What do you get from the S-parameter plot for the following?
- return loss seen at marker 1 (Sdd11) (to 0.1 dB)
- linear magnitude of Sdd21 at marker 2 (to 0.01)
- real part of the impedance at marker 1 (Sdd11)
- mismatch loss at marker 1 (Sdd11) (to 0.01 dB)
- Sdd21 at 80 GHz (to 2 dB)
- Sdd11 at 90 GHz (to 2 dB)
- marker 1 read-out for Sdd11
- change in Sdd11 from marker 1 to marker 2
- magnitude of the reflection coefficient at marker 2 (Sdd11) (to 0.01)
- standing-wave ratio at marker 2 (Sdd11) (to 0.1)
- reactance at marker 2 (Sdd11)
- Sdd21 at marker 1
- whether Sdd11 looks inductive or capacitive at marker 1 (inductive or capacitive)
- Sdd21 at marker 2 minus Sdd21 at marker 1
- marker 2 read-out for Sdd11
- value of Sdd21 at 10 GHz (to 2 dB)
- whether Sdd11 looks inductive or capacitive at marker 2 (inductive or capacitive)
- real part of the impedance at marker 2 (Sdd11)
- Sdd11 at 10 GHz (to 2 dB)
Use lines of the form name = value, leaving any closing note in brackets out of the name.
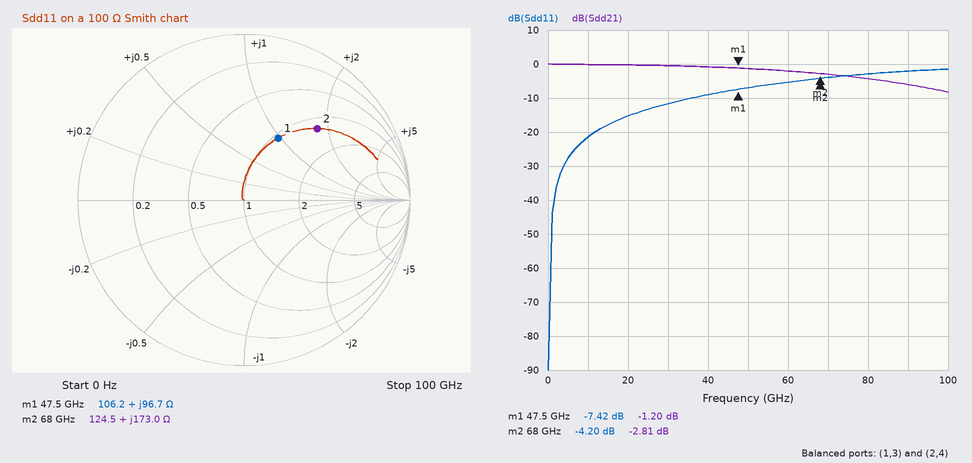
return loss seen at marker 1 (Sdd11) = 7.4 dB
linear magnitude of Sdd21 at marker 2 = 0.72
real part of the impedance at marker 1 = 106.2 Ω
mismatch loss at marker 1 (Sdd11) = 0.87 dB
Sdd21 at 80 GHz = -4 dB
Sdd11 at 90 GHz = -2 dB
marker 1 read-out for Sdd11 = -7.42 dB
change in Sdd11 from marker 1 to marker 2 = 3.22 dB
magnitude of the reflection coefficient at marker 2 (Sdd11) = 0.62
standing-wave ratio at marker 2 (Sdd11) = 4.2
reactance at marker 2 = +173.0 Ω
Sdd21 at marker 1 = -1.20 dB
whether Sdd11 looks inductive or capacitive at marker 1 = inductive
Sdd21 at marker 2 minus Sdd21 at marker 1 = -1.61 dB
marker 2 read-out for Sdd11 = -4.20 dB
value of Sdd21 at 10 GHz = 0 dB
whether Sdd11 looks inductive or capacitive at marker 2 = inductive
real part of the impedance at marker 2 = 124.5 Ω
Sdd11 at 10 GHz = -22 dB
